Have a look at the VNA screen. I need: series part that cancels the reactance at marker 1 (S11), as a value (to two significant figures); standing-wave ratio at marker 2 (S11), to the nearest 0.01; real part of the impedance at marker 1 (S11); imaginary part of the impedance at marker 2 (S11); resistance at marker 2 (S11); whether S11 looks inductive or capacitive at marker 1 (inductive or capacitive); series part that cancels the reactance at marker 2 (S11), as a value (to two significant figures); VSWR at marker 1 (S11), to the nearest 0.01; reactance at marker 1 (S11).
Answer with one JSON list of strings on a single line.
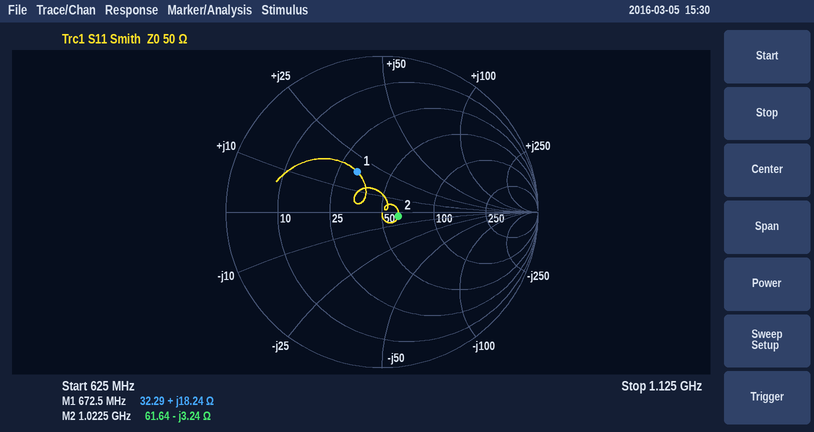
["13 pF", "1.24", "32.29 Ω", "-3.24 Ω", "61.64 Ω", "inductive", "500 pH", "1.86", "+18.24 Ω"]
